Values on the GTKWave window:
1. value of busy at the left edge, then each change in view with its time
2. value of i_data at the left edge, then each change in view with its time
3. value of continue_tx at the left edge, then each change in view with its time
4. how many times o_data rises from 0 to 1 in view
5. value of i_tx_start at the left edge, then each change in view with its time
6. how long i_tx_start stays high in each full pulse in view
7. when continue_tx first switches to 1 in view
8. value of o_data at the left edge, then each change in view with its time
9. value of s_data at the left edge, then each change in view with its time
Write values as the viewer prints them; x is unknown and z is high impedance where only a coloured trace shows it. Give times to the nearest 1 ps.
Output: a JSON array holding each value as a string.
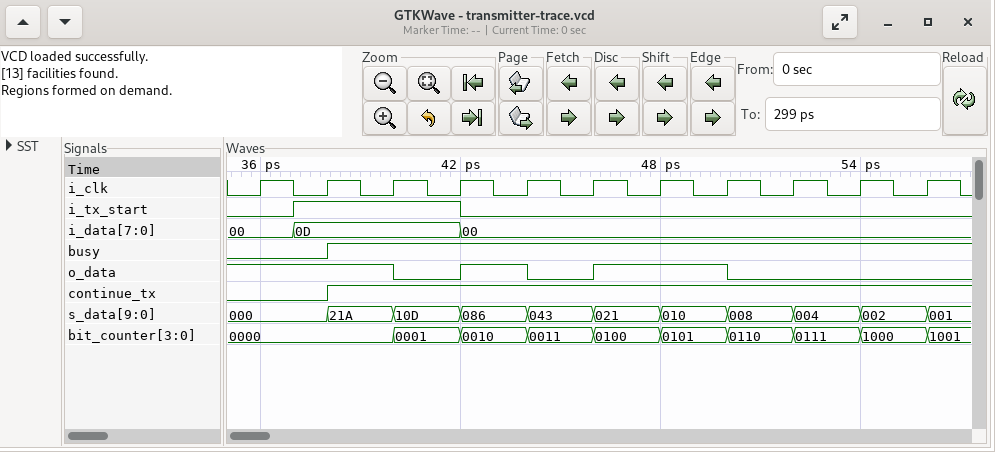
["0, 1 at 38 ps", "00, 0D at 37 ps, 00 at 42 ps", "0, 1 at 38 ps", "2", "0, 1 at 37 ps, 0 at 42 ps", "5 ps", "38 ps", "1, 0 at 40 ps, 1 at 42 ps, 0 at 44 ps, 1 at 46 ps, 0 at 50 ps", "000, 21A at 38 ps, 10D at 40 ps, 086 at 42 ps, 043 at 44 ps, 021 at 46 ps, 010 at 48 ps, 008 at 50 ps, 004 at 52 ps, 002 at 54 ps, 001 at 56 ps"]
